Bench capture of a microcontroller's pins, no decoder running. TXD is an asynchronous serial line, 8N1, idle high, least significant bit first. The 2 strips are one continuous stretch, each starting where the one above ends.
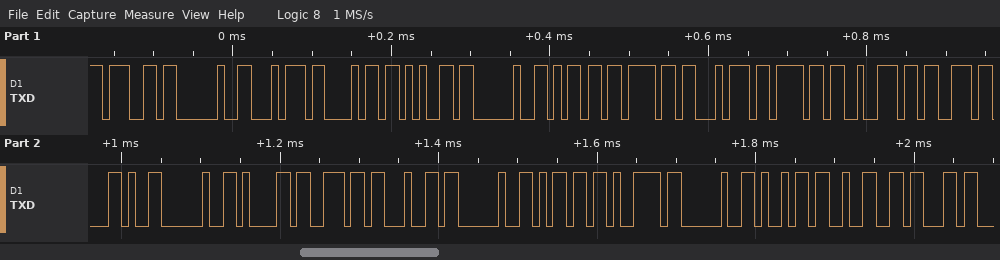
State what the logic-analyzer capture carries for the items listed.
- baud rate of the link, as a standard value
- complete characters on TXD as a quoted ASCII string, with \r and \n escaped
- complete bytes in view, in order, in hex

115200 baud
"g the motors, and my i2c"
0x67 0x20 0x74 0x68 0x65 0x20 0x6D 0x6F 0x74 0x6F 0x72 0x73 0x2C 0x20 0x61 0x6E 0x64 0x20 0x6D 0x79 0x20 0x69 0x32 0x63
